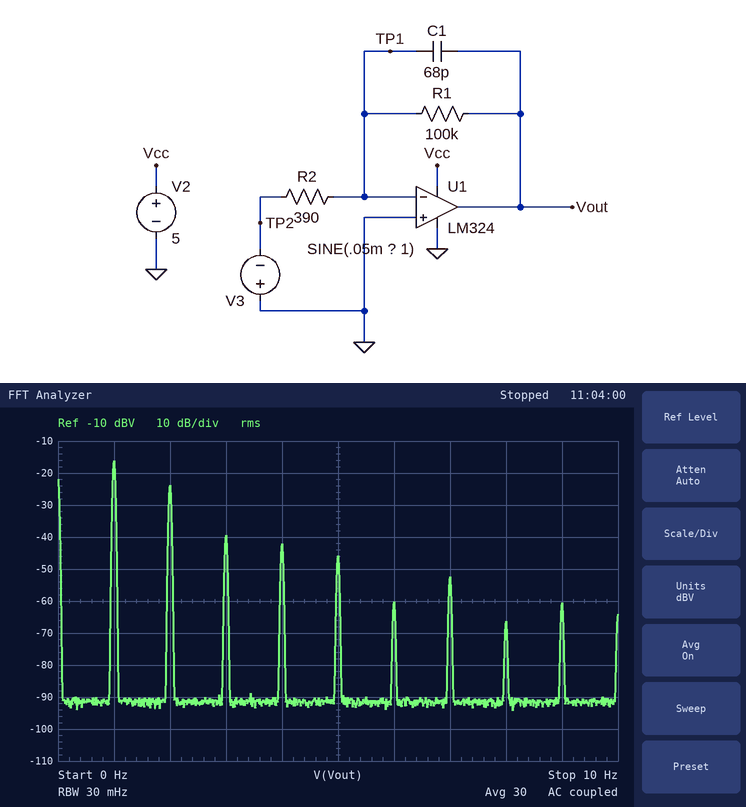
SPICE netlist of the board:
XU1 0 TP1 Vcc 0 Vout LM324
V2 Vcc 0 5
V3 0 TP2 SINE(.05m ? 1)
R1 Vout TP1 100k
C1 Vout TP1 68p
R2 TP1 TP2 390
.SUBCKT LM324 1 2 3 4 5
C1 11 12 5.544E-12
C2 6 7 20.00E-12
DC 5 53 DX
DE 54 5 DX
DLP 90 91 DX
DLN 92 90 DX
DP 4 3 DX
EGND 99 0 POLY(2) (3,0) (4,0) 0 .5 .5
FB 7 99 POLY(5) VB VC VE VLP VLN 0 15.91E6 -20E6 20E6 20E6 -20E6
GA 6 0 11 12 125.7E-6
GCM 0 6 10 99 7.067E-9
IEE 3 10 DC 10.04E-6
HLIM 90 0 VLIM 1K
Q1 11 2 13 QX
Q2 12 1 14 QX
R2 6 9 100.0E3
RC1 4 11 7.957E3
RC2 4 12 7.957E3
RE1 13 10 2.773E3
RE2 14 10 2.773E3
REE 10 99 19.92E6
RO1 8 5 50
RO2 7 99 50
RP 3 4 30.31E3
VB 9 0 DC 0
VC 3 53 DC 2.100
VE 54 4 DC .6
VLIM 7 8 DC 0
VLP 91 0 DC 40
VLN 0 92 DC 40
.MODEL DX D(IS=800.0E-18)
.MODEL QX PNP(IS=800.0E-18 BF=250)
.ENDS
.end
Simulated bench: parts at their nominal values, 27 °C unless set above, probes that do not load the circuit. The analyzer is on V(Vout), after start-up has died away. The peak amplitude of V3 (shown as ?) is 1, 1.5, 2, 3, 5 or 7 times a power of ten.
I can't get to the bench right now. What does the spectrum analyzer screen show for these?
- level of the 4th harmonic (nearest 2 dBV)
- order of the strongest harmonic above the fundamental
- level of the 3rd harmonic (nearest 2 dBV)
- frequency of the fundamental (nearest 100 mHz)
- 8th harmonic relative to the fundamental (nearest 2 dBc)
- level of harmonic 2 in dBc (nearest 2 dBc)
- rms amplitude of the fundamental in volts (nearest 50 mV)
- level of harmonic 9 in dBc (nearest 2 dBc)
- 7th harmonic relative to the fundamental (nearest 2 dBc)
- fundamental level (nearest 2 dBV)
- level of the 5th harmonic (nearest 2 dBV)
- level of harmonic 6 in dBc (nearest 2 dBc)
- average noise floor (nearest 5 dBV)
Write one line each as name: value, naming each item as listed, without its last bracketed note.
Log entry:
level of the 4th harmonic: -42 dBV
order of the strongest harmonic above the fundamental: 2
level of the 3rd harmonic: -40 dBV
frequency of the fundamental: 1.0 Hz
8th harmonic relative to the fundamental: -50 dBc
level of harmonic 2 in dBc: -8 dBc
rms amplitude of the fundamental in volts: 150 mV
level of harmonic 9 in dBc: -44 dBc
7th harmonic relative to the fundamental: -36 dBc
fundamental level: -16 dBV
level of the 5th harmonic: -46 dBV
level of harmonic 6 in dBc: -44 dBc
average noise floor: -90 dBV
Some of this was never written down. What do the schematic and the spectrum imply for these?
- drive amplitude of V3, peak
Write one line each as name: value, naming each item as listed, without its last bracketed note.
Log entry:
drive amplitude of V3, peak: 2 mV
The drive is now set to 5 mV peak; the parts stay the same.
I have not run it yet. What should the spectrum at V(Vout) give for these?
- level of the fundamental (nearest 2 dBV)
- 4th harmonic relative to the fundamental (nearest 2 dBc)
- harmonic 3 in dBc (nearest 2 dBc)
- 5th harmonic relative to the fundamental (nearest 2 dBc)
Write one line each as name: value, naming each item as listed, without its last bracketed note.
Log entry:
level of the fundamental: -8 dBV
4th harmonic relative to the fundamental: -22 dBc
harmonic 3 in dBc: -32 dBc
5th harmonic relative to the fundamental: -36 dBc
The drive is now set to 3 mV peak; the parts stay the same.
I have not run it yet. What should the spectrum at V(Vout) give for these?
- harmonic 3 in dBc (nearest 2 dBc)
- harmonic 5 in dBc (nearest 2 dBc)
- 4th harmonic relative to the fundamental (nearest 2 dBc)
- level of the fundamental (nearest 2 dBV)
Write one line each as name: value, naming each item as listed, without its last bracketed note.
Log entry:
harmonic 3 in dBc: -28 dBc
harmonic 5 in dBc: -32 dBc
4th harmonic relative to the fundamental: -24 dBc
level of the fundamental: -12 dBV
